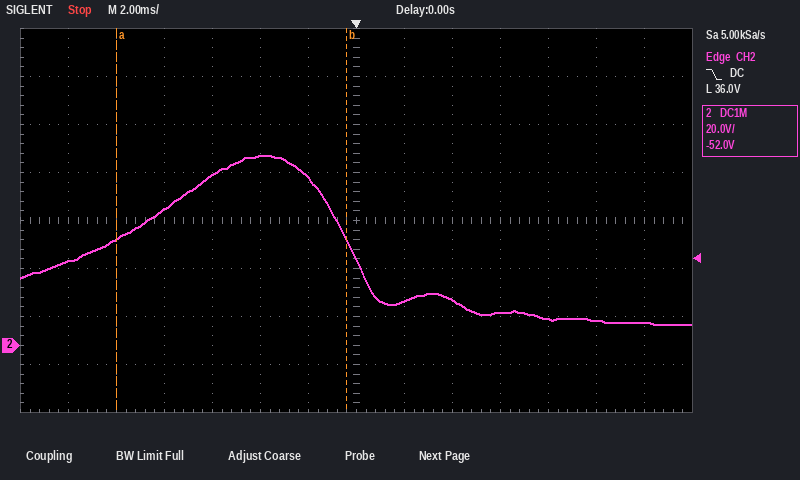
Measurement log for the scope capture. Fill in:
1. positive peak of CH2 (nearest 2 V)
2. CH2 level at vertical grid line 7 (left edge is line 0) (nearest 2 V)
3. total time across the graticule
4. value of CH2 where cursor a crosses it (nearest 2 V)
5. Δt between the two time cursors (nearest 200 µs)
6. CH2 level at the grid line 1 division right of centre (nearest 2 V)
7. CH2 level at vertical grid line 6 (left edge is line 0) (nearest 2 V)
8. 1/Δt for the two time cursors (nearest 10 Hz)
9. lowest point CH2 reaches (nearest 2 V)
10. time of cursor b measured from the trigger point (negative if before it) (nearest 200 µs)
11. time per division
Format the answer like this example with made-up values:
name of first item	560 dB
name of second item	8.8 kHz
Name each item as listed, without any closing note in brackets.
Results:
positive peak of CH2	80 V
CH2 level at vertical grid line 7 (left edge is line 0)	36 V
total time across the graticule	28 ms
value of CH2 where cursor a crosses it	44 V
Δt between the two time cursors	9.6 ms
CH2 level at the grid line 1 division right of centre	18 V
CH2 level at vertical grid line 6 (left edge is line 0)	70 V
1/Δt for the two time cursors	100 Hz
lowest point CH2 reaches	8 V
time of cursor b measured from the trigger point (negative if before it)	-400 µs
time per division	2 ms
